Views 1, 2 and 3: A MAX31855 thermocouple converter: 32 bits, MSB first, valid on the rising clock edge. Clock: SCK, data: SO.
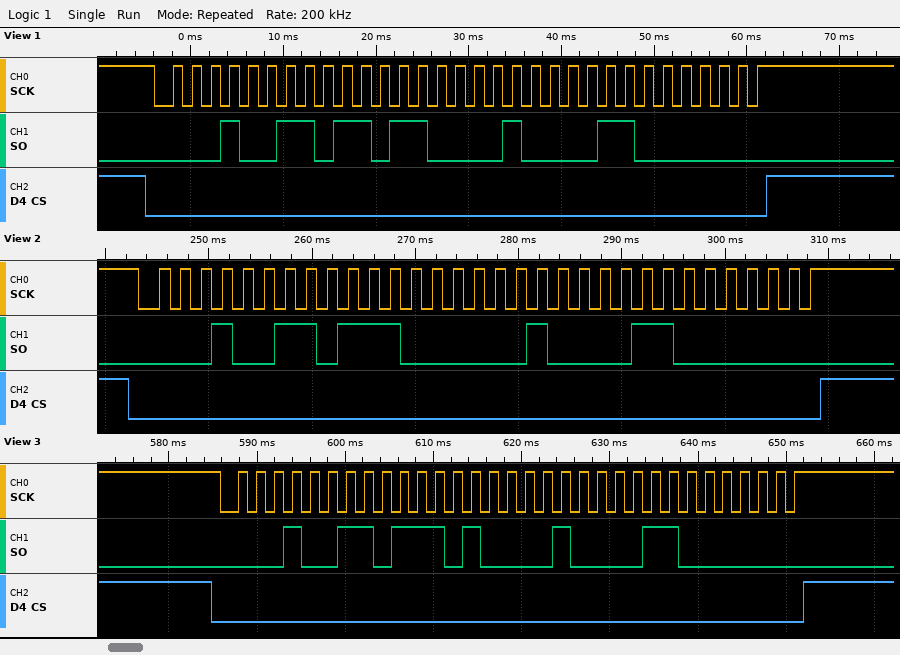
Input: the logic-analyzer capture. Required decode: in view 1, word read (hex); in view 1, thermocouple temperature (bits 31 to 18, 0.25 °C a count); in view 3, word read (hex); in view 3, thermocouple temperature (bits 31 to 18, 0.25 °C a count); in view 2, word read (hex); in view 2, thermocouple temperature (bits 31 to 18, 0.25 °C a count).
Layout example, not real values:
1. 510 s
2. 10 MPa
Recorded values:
1. 0x136C2180
2. 310.75 °C
3. 0x13742180
4. 311.25 °C
5. 0x13702180
6. 311.00 °C
